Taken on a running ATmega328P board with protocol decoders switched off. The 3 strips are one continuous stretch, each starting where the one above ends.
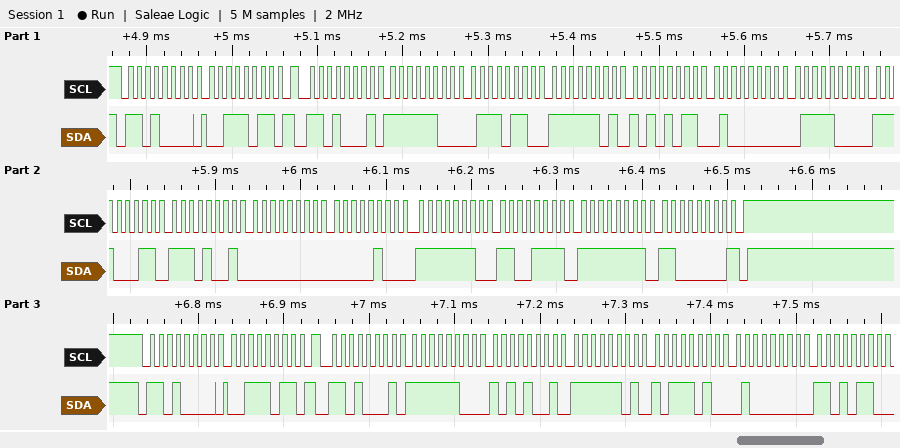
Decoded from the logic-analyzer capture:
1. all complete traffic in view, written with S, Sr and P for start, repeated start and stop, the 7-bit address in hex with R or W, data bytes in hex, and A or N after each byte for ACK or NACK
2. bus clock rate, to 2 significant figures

S 68W A 3B A Sr 68R A FC A 76 A FD A AB A 40 A 78 A E3 A E9 A 00 A 04 A FE A CF A FF A C0 N P S 68W A 3B A Sr 68R A FC A A9 A FD A BA A 40 A D6 A
100 kHz
